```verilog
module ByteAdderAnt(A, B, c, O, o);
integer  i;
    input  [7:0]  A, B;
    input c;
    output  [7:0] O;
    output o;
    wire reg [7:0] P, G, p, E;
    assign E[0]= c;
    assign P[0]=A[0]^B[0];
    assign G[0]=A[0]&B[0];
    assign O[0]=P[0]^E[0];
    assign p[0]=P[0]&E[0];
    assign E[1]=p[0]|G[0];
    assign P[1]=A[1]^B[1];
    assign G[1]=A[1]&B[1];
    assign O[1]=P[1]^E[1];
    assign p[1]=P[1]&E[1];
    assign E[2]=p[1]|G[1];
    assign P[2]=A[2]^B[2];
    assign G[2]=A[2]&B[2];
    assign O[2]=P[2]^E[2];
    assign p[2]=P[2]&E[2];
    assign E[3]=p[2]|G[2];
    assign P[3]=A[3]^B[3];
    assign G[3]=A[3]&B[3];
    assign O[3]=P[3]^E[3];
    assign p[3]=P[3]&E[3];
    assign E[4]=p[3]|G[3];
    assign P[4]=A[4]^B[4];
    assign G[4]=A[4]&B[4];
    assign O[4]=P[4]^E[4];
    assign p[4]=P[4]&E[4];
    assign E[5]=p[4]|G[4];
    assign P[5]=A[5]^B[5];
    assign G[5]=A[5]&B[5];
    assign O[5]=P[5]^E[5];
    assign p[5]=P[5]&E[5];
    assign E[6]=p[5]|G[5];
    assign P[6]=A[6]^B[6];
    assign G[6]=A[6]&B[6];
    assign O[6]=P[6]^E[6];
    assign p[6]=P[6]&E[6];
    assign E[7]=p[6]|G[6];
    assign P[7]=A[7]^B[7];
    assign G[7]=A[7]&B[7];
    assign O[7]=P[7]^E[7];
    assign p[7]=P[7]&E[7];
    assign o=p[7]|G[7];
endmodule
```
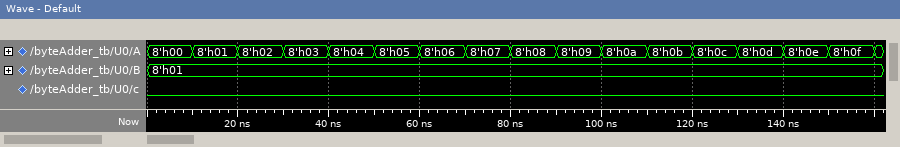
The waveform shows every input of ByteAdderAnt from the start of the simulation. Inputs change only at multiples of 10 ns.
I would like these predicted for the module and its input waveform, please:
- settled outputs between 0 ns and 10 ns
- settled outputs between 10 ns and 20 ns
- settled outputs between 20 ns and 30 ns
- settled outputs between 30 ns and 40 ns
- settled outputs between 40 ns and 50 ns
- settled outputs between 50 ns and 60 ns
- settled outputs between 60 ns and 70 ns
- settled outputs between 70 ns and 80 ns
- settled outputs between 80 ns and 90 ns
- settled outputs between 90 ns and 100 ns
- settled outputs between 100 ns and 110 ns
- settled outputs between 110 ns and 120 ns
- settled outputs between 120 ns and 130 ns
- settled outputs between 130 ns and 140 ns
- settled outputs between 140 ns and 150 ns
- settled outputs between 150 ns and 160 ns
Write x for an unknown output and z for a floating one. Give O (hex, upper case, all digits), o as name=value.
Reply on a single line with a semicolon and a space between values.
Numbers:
O=01, o=0; O=02, o=0; O=03, o=0; O=04, o=0; O=05, o=0; O=06, o=0; O=07, o=0; O=08, o=0; O=09, o=0; O=0A, o=0; O=0B, o=0; O=0C, o=0; O=0D, o=0; O=0E, o=0; O=0F, o=0; O=10, o=0
